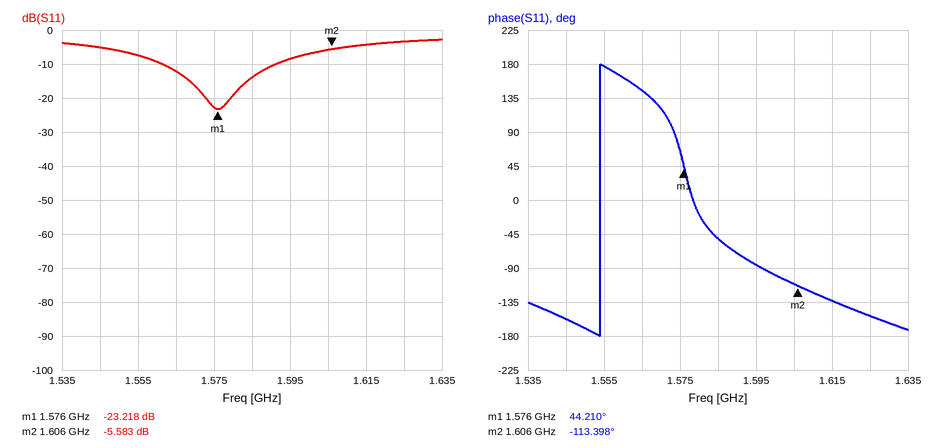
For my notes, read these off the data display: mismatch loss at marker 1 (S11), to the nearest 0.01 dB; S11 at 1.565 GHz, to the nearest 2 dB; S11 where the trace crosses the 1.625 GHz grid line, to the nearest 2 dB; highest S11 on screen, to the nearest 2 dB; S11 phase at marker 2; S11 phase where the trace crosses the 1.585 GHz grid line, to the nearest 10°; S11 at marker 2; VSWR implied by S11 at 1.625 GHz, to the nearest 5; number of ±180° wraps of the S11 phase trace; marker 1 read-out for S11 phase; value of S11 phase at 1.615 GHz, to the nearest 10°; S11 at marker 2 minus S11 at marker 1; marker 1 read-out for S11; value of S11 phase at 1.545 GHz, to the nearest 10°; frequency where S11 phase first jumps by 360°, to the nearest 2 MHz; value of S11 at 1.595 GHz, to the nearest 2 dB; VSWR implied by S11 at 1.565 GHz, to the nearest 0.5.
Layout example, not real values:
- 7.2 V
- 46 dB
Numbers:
- 0.02 dB
- -12 dB
- -4 dB
- -2 dB
- -113.398°
- -50°
- -5.583 dB
- 5
- 1
- 44.210°
- -130°
- 17.635 dB
- -23.218 dB
- -160°
- 1.554 GHz
- -8 dB
- 1.5
